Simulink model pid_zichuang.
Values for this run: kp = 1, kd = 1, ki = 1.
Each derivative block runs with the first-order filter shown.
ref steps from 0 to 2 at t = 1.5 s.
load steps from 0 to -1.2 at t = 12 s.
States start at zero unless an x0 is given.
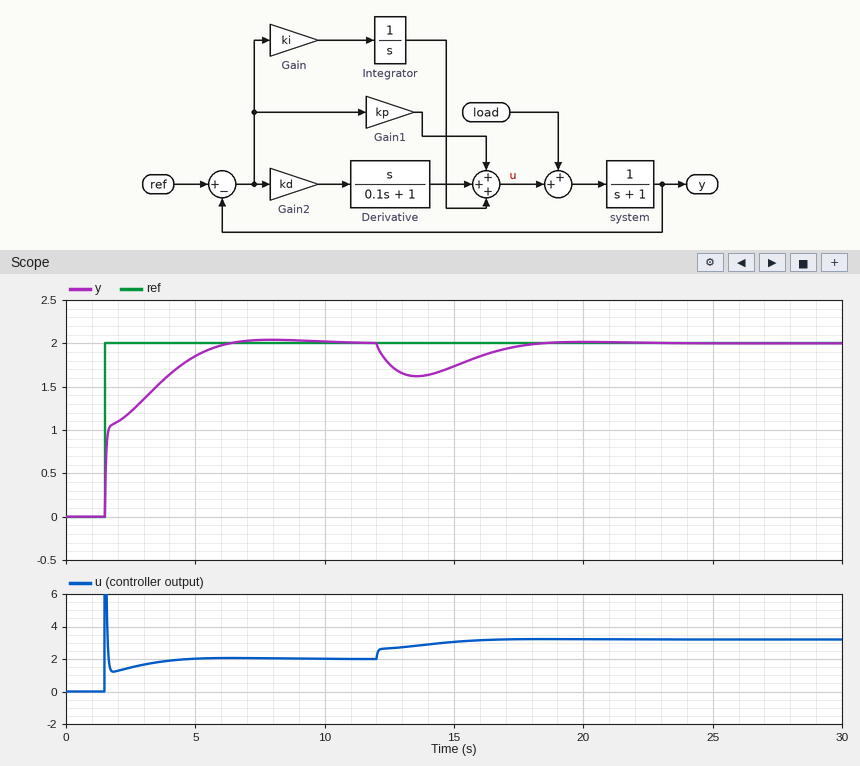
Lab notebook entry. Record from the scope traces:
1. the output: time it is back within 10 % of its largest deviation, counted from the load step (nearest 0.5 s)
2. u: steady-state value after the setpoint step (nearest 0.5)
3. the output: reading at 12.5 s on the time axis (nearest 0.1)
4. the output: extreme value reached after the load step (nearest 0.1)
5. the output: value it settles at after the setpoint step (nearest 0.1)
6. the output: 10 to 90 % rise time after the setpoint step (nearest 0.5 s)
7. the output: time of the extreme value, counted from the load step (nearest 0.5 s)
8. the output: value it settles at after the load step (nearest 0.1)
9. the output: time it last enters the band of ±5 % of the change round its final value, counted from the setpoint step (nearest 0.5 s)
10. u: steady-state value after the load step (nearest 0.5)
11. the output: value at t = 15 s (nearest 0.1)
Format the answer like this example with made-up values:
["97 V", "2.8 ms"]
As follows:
["5.5 s", "2.0", "1.8", "1.6", "2.0", "3.0 s", "1.5 s", "2.0", "4.0 s", "3.0", "1.7"]
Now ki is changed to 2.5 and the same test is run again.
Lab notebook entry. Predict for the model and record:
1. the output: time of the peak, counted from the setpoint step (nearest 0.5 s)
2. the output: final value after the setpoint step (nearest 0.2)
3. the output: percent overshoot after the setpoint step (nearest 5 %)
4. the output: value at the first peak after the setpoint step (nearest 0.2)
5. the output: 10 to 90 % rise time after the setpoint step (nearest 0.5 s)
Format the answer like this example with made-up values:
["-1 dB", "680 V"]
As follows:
["3.0 s", "2.0", "10 %", "2.2", "1.5 s"]
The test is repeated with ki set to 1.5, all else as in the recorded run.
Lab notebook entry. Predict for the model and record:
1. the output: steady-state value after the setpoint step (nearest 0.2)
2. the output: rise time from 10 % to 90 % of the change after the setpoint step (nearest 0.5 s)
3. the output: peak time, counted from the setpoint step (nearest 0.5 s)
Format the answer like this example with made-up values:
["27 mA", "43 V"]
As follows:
["2.0", "2.5 s", "4.5 s"]
